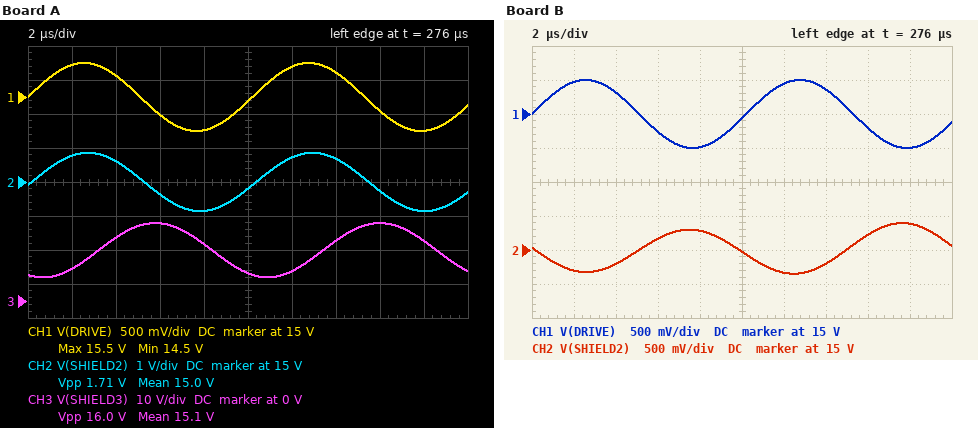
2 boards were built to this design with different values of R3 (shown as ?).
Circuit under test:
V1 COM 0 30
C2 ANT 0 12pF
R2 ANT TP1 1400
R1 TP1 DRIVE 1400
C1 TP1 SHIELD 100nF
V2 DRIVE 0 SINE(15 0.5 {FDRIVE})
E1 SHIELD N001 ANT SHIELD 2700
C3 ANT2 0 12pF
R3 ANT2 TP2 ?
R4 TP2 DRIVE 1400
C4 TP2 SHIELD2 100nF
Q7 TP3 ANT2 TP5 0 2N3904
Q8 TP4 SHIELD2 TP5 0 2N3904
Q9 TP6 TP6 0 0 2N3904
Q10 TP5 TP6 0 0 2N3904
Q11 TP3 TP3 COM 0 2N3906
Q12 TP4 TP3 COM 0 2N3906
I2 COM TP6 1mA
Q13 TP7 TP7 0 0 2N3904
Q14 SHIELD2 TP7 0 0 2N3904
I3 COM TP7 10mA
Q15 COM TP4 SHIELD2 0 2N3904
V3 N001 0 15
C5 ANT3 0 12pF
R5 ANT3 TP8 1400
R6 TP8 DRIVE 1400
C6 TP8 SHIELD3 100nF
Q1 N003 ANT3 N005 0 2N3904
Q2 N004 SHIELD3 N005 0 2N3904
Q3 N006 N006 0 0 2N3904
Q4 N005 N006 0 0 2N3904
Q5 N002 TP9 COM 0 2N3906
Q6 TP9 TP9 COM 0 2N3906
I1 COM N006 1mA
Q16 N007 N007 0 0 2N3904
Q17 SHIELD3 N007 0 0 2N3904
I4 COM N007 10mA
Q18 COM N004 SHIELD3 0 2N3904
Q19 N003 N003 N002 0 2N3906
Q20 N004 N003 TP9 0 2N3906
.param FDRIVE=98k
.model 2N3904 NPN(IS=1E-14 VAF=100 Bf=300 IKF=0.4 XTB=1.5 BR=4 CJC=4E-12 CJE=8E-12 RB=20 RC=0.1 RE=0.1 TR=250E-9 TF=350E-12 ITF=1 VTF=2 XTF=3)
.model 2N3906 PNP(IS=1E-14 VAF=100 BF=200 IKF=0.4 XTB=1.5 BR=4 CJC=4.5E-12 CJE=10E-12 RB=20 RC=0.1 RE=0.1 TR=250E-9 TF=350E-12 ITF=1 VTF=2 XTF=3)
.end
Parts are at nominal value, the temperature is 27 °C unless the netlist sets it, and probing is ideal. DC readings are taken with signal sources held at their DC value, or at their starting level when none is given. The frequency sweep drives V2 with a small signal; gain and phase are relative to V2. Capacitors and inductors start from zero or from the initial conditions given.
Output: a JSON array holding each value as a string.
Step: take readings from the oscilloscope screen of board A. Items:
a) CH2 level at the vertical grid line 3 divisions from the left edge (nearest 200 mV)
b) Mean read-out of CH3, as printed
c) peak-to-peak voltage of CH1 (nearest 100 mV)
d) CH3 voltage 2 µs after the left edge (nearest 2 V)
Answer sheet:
["14.6 V", "15.1 V", "1.0 V", "10 V"]
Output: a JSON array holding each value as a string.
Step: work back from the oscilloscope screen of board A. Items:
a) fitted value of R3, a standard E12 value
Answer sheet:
["560 Ω"]
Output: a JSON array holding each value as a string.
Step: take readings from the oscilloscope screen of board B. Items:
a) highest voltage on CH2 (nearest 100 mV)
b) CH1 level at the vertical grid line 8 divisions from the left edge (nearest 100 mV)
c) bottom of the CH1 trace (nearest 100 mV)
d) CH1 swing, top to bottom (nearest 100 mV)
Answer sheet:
["15.4 V", "14.8 V", "14.5 V", "1.0 V"]
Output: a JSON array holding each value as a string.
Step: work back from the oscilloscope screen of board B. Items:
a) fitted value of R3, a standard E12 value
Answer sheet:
["3.3 kΩ"]
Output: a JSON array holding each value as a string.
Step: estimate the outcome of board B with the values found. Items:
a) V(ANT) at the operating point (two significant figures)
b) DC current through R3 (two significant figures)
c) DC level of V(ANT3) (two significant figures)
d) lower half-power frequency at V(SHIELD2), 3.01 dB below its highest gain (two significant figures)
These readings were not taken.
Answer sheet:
["15 V", "1.6 µA", "15 V", "61 kHz"]
